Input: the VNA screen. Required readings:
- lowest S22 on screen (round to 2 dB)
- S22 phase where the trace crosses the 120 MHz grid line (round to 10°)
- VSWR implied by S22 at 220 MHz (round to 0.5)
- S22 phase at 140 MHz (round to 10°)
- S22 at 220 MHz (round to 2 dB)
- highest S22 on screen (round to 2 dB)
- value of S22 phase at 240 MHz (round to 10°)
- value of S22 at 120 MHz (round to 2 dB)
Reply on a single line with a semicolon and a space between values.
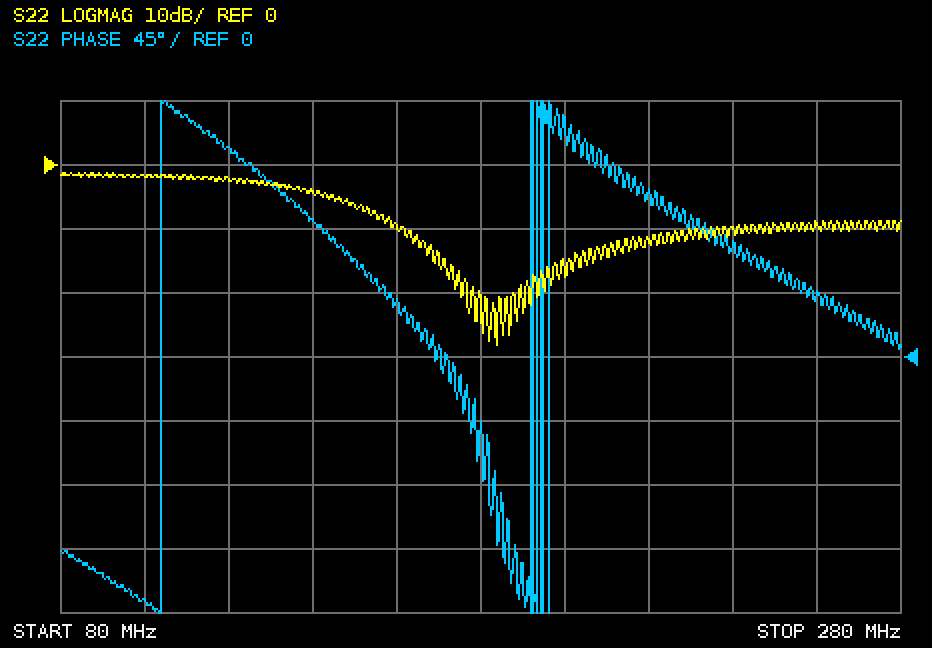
-28 dB; 150°; 1.5; 100°; -12 dB; -2 dB; 80°; -2 dB
